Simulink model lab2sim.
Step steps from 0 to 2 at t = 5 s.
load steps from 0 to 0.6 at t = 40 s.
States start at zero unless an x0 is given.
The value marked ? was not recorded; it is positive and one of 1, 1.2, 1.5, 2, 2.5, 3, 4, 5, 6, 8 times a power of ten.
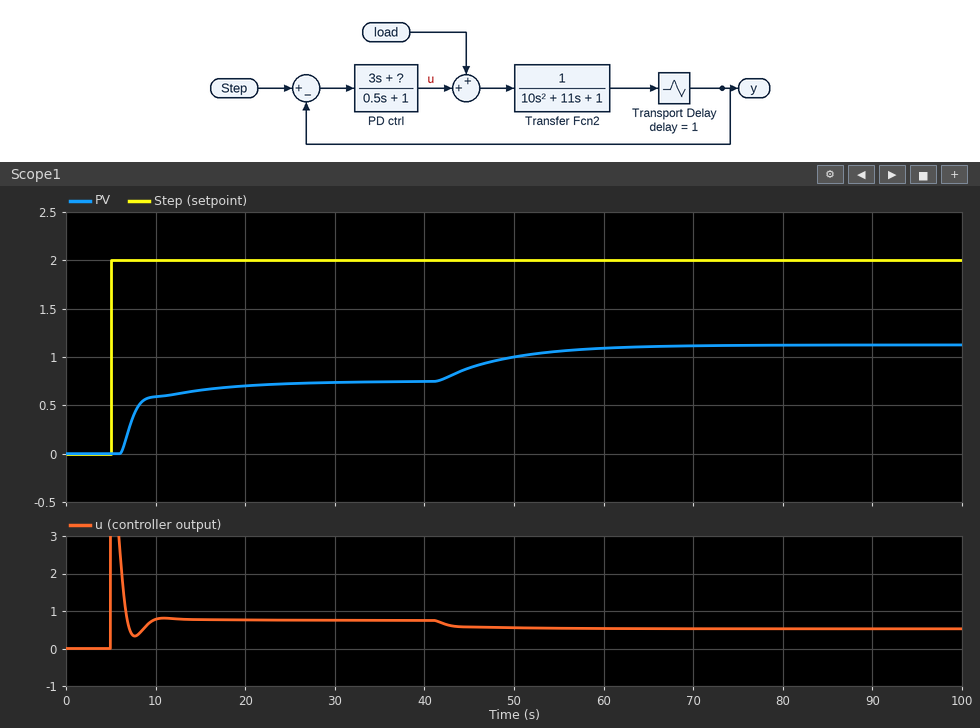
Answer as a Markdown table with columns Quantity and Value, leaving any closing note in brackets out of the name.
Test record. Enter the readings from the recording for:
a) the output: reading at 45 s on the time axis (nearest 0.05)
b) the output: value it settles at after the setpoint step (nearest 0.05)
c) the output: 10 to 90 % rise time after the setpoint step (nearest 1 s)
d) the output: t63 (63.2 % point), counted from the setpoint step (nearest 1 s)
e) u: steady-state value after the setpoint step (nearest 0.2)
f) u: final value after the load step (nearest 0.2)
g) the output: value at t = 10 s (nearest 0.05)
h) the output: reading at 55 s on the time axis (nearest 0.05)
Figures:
| Quantity | Value |
|---|---|
| the output: reading at 45 s on the time axis | 0.90 |
| the output: value it settles at after the setpoint step | 0.75 |
| the output: 10 to 90 % rise time after the setpoint step | 10 s |
| the output: t63 (63.2 % point), counted from the setpoint step | 3 s |
| u: steady-state value after the setpoint step | 0.8 |
| u: final value after the load step | 0.6 |
| the output: value at t = 10 s | 0.60 |
| the output: reading at 55 s on the time axis | 1.05 |
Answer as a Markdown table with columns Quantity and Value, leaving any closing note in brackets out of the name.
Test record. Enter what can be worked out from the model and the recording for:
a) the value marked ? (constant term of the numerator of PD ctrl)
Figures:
| Quantity | Value |
|---|---|
| the value marked ? | 0.6 |
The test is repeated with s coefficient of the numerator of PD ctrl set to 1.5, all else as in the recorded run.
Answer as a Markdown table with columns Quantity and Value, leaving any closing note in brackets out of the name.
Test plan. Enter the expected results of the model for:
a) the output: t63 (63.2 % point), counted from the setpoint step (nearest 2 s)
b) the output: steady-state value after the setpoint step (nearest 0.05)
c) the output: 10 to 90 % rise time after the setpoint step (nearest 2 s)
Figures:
| Quantity | Value |
|---|---|
| the output: t63 (63.2 % point), counted from the setpoint step | 6 s |
| the output: steady-state value after the setpoint step | 0.75 |
| the output: 10 to 90 % rise time after the setpoint step | 12 s |
